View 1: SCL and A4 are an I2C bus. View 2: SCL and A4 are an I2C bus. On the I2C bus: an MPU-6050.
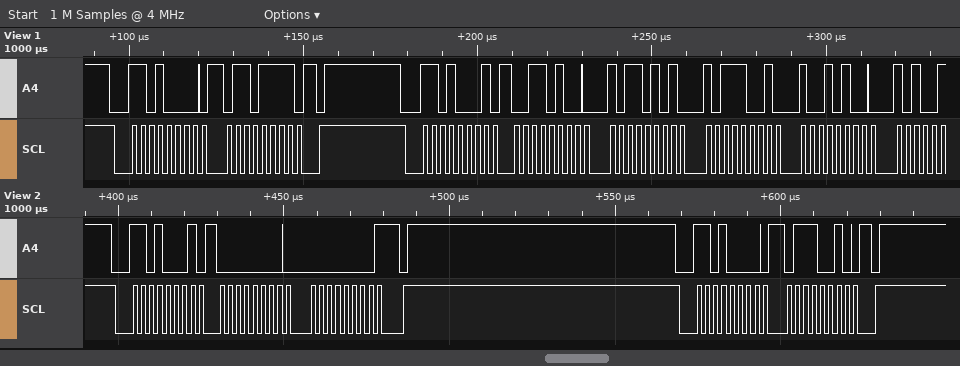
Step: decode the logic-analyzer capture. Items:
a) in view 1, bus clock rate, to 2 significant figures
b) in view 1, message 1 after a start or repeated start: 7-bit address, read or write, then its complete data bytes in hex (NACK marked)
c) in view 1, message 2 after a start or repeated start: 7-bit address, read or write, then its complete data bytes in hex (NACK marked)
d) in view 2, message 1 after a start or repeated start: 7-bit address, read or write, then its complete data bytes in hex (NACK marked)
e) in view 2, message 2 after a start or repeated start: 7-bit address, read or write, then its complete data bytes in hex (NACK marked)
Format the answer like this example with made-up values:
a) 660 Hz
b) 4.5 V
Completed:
a) 400 kHz
b) 0x68 write: 6F
c) 0x68 read: 34 B5 B9 94
d) 0x68 read: 00 00 NACK
e) 0x68 write: 72
